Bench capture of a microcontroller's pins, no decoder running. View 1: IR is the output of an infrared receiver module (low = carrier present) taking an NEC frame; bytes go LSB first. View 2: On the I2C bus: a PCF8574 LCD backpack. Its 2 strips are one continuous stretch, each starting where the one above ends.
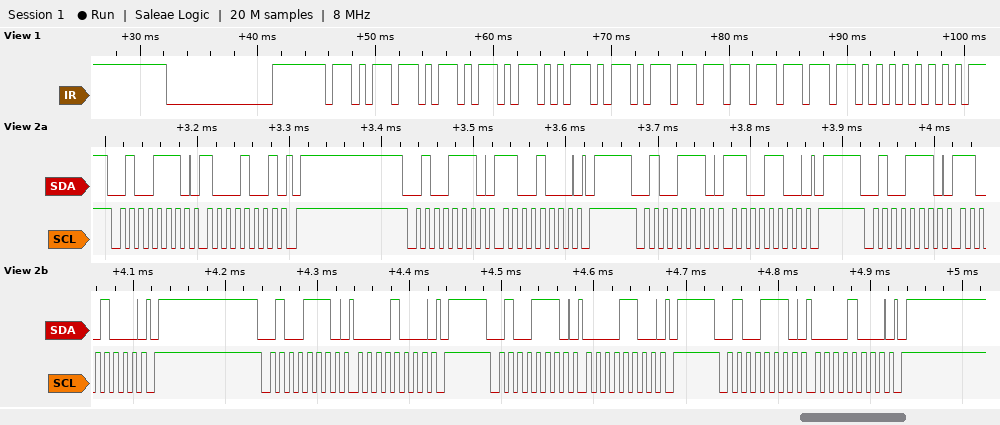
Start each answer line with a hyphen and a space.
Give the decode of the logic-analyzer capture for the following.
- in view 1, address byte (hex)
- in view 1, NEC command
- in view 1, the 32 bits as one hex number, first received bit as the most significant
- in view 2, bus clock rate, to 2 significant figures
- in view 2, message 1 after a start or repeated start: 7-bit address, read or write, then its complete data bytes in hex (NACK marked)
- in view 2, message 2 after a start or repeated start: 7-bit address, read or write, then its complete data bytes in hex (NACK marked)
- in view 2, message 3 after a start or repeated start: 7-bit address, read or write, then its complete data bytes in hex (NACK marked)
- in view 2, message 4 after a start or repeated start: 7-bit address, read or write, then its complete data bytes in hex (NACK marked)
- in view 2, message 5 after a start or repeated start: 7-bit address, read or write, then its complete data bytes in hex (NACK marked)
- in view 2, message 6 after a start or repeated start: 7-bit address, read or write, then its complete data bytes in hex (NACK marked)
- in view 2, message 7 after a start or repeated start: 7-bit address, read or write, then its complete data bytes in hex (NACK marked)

- 0xAD
- 0xFF
- 0xB54AFF00
- 100 kHz
- 0x27 write: 89
- 0x27 write: C8
- 0x27 write: CC
- 0x27 write: C8
- 0x27 write: 08
- 0x27 write: 0C
- 0x27 write: 08
